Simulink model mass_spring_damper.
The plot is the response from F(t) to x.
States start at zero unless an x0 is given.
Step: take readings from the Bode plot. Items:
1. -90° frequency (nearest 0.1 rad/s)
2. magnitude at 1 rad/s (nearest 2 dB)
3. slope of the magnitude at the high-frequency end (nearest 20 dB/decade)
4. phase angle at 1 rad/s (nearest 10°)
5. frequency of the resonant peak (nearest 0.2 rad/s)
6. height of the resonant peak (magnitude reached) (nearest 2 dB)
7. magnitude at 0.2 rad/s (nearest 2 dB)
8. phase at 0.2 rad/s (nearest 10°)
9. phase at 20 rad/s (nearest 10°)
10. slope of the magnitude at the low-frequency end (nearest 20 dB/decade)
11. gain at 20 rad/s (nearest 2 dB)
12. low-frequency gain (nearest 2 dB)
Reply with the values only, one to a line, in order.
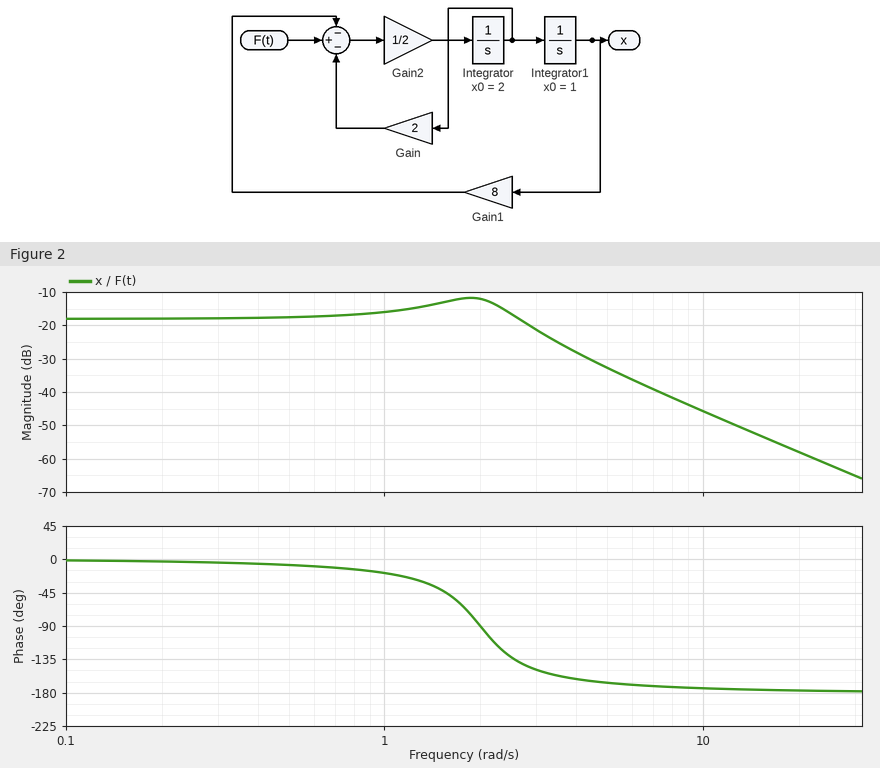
2.0 rad/s
-16 dB
-40 dB/decade
-20°
1.8 rad/s
-12 dB
-18 dB
0°
-180°
0 dB/decade
-58 dB
-18 dB
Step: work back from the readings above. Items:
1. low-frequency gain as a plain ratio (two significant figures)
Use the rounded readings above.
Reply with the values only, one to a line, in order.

0.13
